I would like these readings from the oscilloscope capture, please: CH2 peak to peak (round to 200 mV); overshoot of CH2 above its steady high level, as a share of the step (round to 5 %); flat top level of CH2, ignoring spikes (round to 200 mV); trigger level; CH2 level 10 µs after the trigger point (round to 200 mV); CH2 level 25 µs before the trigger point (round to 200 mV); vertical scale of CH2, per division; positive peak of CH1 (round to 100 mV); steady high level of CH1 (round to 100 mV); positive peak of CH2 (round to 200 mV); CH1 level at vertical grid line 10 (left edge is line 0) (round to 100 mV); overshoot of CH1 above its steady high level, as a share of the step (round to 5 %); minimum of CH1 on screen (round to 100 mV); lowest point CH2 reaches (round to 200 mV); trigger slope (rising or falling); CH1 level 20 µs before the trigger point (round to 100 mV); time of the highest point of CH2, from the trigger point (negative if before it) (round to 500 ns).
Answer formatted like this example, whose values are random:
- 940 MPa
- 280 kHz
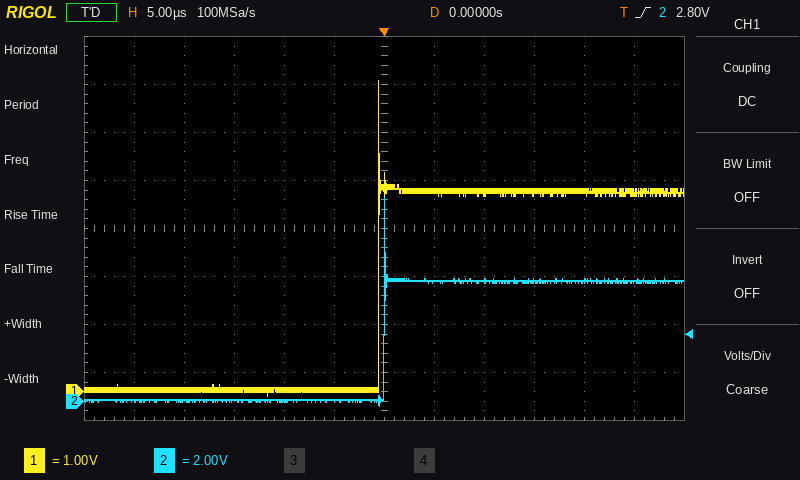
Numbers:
- 8.6 V
- 70 %
- 5.0 V
- 2.80 V
- 5.0 V
- 0.0 V
- 2 V
- 6.5 V
- 4.2 V
- 8.4 V
- 4.2 V
- 55 %
- -100 mV
- -200 mV
- rising
- 0.0 V
- 0.0 µs
